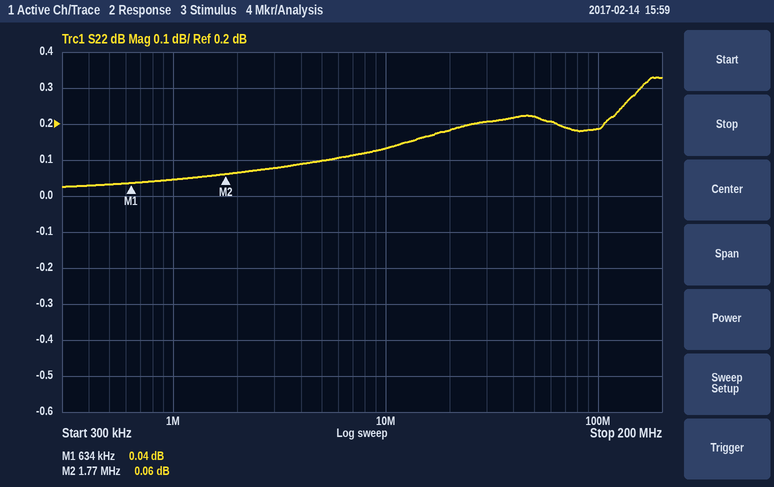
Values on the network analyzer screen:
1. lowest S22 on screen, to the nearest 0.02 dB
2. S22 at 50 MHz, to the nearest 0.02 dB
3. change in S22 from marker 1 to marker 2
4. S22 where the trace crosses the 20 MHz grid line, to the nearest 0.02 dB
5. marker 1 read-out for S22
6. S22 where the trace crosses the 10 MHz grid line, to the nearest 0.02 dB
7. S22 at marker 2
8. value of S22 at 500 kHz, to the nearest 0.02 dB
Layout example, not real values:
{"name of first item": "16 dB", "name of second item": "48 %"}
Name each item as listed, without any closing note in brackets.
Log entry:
{"lowest S22 on screen, to the nearest 0.02 dB": "0.02 dB", "S22 at 50 MHz, to the nearest 0.02 dB": "0.22 dB", "change in S22 from marker 1 to marker 2": "0.02 dB", "S22 where the trace crosses the 20 MHz grid line, to the nearest 0.02 dB": "0.18 dB", "marker 1 read-out for S22": "0.04 dB", "S22 where the trace crosses the 10 MHz grid line, to the nearest 0.02 dB": "0.14 dB", "S22 at marker 2": "0.06 dB", "value of S22 at 500 kHz, to the nearest 0.02 dB": "0.04 dB"}
